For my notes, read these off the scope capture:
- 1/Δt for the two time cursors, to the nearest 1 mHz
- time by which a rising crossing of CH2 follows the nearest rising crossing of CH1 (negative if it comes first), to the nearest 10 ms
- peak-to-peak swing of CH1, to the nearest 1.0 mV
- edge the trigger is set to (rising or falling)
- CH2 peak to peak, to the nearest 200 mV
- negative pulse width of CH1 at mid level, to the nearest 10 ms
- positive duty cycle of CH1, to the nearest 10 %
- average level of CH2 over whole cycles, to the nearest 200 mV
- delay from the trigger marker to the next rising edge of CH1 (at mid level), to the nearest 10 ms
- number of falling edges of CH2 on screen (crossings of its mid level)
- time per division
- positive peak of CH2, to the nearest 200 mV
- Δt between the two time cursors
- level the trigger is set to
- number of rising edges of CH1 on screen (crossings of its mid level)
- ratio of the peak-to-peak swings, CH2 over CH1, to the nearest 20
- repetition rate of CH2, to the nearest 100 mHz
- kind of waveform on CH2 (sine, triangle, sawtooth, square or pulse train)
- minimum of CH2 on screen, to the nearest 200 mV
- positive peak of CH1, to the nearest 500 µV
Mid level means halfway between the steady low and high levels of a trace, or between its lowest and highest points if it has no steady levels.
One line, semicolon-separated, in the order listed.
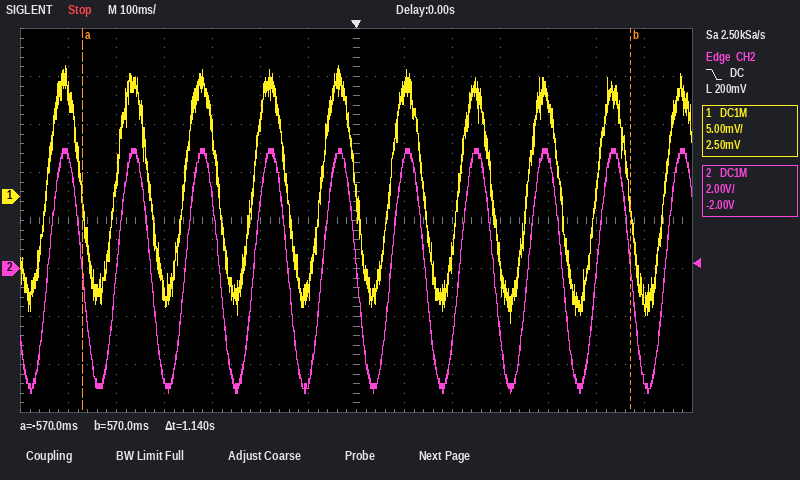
877 mHz; 0 ms; 27.0 mV; falling; 10.2 V; 70 ms; 50 %; 0.0 V; 70 ms; 9; 100 ms; 5.0 V; 1.14 s; 200 mV; 10; 380; 7.0 Hz; sine; -5.2 V; 13.5 mV
